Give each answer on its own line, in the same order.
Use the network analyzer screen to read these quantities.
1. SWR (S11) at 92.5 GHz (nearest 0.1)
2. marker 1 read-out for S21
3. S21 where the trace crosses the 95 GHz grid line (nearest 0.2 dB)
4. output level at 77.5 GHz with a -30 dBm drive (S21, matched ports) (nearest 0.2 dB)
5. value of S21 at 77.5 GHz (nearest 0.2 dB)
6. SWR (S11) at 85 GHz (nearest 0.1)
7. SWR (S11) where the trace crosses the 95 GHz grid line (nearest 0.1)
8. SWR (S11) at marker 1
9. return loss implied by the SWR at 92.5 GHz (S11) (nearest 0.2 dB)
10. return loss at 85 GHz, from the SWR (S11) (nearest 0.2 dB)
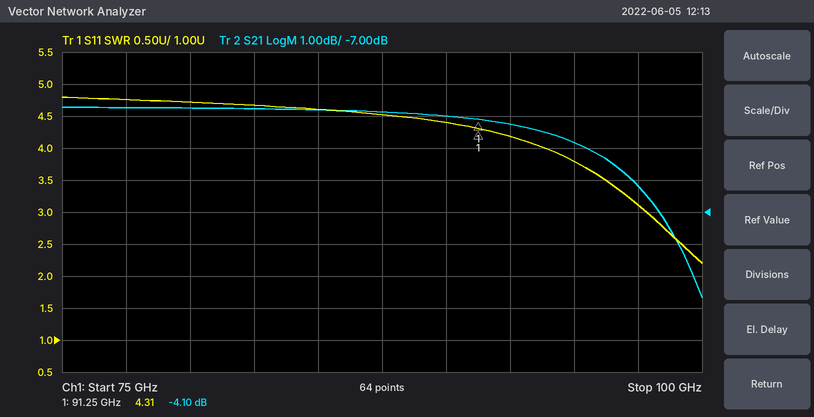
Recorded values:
4.2
-4.10 dB
-4.8 dB
-33.8 dBm
-3.8 dB
4.6
3.8
4.31
4.2 dB
3.8 dB
